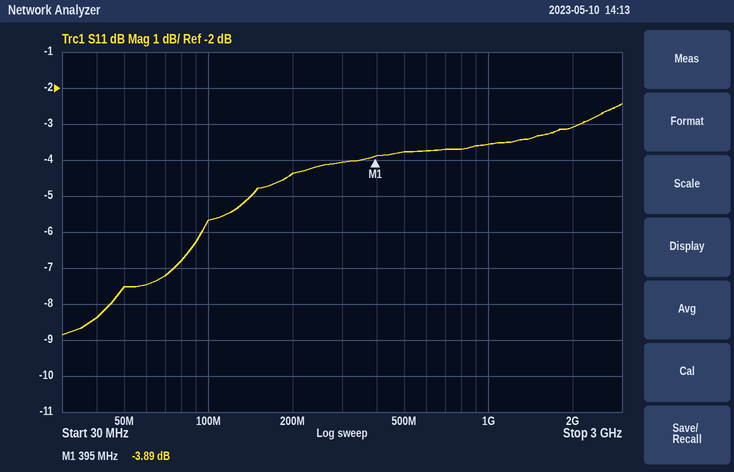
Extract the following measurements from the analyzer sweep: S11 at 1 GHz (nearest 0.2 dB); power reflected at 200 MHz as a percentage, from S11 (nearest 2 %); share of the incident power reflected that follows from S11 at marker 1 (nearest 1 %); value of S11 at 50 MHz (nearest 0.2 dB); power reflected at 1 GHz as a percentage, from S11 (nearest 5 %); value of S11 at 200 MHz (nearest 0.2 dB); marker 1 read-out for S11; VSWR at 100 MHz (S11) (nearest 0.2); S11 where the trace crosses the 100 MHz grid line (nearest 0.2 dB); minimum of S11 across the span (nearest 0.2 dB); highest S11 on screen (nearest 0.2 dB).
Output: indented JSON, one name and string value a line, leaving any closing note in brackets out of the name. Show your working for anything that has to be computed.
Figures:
{
  "S11 at 1 GHz": "-3.6 dB",
  "power reflected at 200 MHz as a percentage, from S11": "10^(-4.4/10) ≈ 36 %",
  "share of the incident power reflected that follows from S11 at marker 1": "10^(-3.89/10) ≈ 41 %",
  "value of S11 at 50 MHz": "-7.6 dB",
  "power reflected at 1 GHz as a percentage, from S11": "10^(-3.6/10) ≈ 43.7 %, so 45 % to the nearest 5 %",
  "value of S11 at 200 MHz": "-4.4 dB",
  "marker 1 read-out for S11": "-3.89 dB",
  "VSWR at 100 MHz (S11)": "|Γ| = 10^(-5.6/20) = 0.5248; VSWR = (1 + 0.5248)/(1 − 0.5248) ≈ 3.2",
  "S11 where the trace crosses the 100 MHz grid line": "-5.6 dB",
  "minimum of S11 across the span": "-8.8 dB",
  "highest S11 on screen": "-2.4 dB"
}
